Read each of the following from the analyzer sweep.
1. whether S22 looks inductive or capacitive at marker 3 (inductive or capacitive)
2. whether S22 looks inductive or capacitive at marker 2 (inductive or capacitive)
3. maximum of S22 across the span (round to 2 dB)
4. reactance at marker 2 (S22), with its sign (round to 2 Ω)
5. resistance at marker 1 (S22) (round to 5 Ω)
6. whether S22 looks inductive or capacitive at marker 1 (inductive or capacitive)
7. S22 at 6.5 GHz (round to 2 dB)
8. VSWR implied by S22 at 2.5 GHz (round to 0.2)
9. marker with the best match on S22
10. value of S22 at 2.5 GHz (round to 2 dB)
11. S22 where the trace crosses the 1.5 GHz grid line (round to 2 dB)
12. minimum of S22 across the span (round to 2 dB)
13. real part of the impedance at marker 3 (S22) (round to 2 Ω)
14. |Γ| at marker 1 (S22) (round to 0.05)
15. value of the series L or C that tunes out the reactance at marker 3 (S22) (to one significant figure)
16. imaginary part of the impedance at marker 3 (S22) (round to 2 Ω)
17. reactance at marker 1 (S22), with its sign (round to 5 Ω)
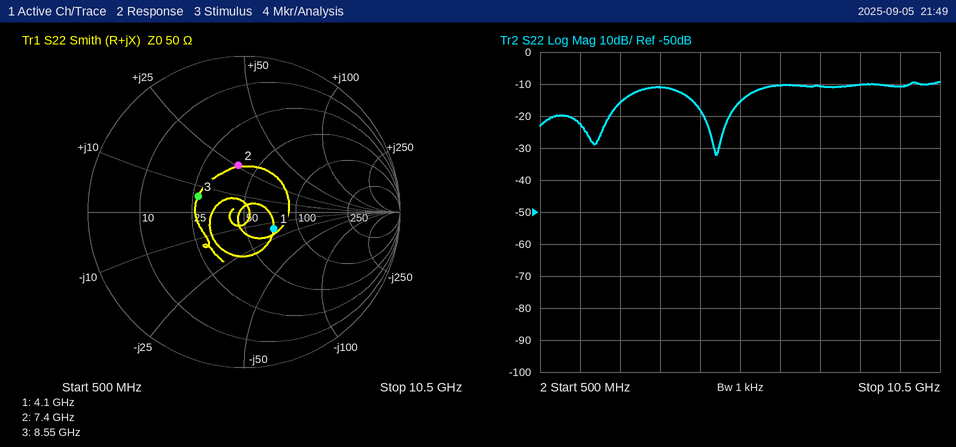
inductive
inductive
-10 dB
+26 Ω
70 Ω
capacitive
-10 dB
1.4
marker 1
-16 dB
-22 dB
-32 dB
26 Ω
0.20
3 pF
+6 Ω
-15 Ω
